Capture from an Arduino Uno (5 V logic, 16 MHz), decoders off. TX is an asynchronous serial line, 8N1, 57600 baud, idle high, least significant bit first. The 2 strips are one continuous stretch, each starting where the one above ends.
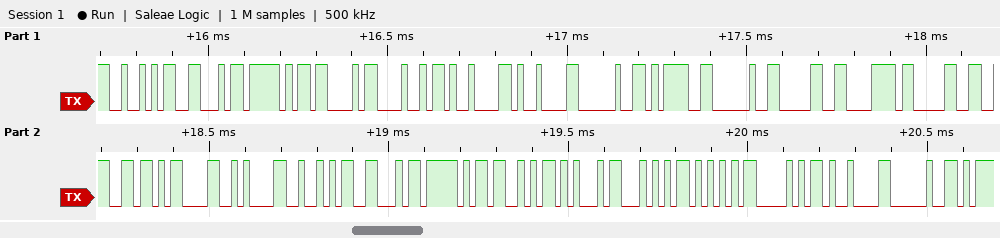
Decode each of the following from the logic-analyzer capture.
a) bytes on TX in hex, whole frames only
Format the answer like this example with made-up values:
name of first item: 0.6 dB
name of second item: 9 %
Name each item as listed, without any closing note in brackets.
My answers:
bytes on TX in hex, whole frames only: 52 46 5F 43 48 09 09 20 3D 20 30 78 30 66 0D 0A 52 46 5F 53 45 54 55 50 09 20
